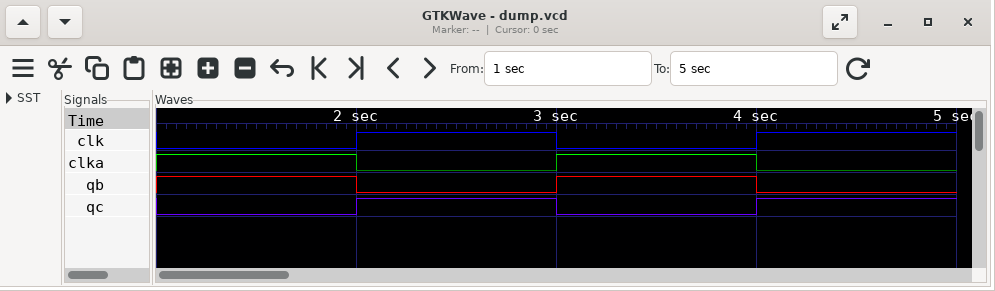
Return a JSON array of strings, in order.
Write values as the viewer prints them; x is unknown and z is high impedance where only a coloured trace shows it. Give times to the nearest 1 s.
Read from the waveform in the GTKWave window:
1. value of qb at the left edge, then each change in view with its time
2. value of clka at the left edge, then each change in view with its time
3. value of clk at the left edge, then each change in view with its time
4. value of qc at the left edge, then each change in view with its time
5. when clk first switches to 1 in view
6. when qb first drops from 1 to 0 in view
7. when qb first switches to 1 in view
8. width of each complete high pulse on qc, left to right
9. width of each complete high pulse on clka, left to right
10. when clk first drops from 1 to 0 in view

["1, 0 at 2 s, 1 at 3 s, 0 at 4 s", "1, 0 at 2 s, 1 at 3 s, 0 at 4 s", "0, 1 at 2 s, 0 at 3 s, 1 at 4 s", "0, 1 at 2 s, 0 at 3 s, 1 at 4 s", "2 s", "2 s", "3 s", "1 s", "1 s", "3 s"]
